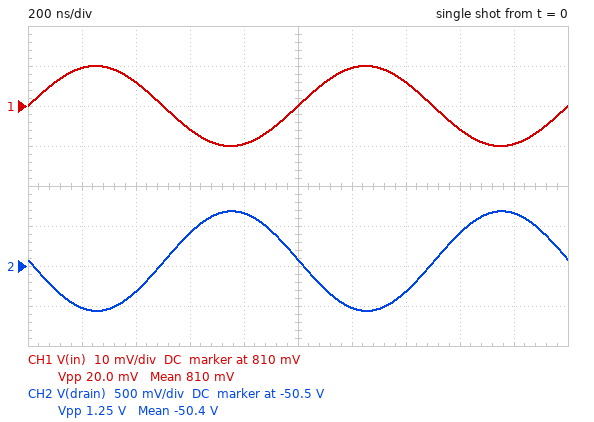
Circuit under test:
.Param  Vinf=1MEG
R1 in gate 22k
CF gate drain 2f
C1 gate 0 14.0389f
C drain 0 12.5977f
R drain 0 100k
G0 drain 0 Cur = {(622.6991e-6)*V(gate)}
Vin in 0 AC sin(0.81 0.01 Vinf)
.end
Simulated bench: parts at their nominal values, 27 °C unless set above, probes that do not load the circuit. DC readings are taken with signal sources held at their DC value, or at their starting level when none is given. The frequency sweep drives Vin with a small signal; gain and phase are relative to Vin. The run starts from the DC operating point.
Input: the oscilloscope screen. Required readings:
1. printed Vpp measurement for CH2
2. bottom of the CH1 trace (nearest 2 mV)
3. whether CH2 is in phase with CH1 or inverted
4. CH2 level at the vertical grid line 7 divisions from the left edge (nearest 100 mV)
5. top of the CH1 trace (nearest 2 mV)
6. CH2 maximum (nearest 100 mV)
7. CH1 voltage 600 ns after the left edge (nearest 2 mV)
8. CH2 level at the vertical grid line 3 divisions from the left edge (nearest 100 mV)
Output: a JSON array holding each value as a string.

["1.25 V", "800 mV", "inverted", "-50.8 V", "820 mV", "-49.8 V", "804 mV", "-50.1 V"]
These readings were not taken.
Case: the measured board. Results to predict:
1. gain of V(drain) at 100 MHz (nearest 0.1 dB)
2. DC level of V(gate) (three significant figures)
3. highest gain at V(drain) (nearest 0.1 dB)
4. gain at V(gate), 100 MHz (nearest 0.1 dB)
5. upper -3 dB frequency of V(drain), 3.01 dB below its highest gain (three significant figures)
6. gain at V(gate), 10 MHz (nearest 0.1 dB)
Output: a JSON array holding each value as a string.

["26.4 dB", "810 mV", "35.9 dB", "-6.8 dB", "35.8 MHz", "-0.3 dB"]
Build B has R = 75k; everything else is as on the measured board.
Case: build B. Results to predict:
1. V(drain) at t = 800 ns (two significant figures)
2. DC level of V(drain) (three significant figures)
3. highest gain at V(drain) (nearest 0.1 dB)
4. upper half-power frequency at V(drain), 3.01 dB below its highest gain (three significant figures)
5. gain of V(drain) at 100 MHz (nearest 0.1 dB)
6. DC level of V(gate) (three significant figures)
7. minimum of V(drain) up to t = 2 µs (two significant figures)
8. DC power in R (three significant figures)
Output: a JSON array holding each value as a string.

["-37 V", "-37.8 V", "33.4 dB", "46.9 MHz", "25.9 dB", "810 mV", "-38 V", "19.1 mW"]
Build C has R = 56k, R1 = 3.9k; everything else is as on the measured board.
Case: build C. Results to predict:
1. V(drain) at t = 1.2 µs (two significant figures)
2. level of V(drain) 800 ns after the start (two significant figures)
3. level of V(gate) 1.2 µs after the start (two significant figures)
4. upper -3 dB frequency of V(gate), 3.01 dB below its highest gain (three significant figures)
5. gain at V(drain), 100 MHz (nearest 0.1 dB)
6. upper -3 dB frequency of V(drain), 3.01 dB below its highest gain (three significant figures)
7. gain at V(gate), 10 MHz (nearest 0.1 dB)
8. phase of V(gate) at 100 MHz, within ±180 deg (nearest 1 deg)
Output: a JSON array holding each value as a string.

["-29 V", "-28 V", "820 mV", "1.14 GHz", "29.1 dB", "144 MHz", "0 dB", "-9 deg"]
